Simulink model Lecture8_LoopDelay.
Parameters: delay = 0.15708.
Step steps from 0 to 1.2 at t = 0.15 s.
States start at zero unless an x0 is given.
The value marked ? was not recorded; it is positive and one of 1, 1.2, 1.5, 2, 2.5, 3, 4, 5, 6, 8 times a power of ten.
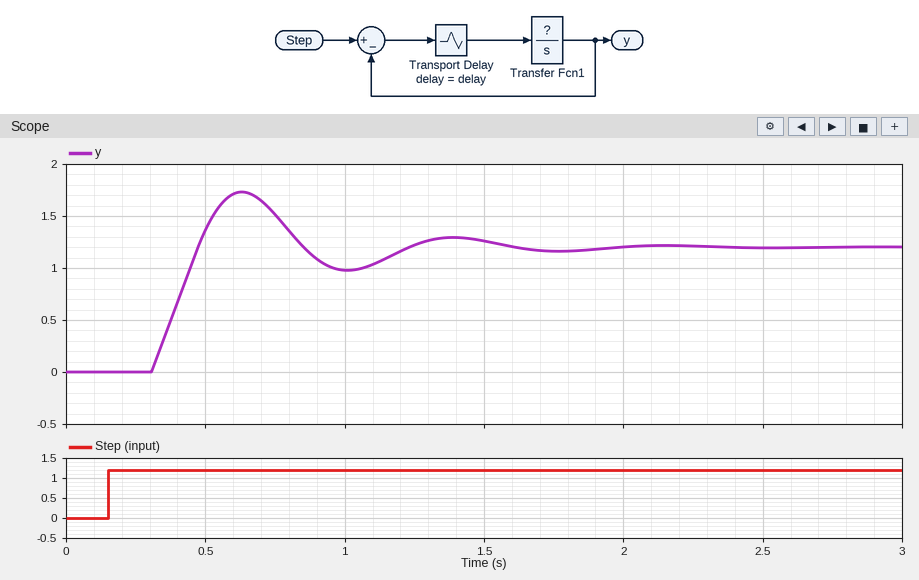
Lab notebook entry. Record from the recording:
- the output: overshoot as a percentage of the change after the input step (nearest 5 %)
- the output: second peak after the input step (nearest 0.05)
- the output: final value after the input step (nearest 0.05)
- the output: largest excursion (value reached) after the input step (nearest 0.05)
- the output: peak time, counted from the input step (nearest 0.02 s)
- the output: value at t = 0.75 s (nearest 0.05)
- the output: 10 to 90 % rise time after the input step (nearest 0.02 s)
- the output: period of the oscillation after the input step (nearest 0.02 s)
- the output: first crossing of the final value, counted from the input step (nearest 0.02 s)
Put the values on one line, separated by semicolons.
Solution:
45 %; 1.30; 1.20; 1.75; 0.48 s; 1.50; 0.14 s; 0.76 s; 0.32 s
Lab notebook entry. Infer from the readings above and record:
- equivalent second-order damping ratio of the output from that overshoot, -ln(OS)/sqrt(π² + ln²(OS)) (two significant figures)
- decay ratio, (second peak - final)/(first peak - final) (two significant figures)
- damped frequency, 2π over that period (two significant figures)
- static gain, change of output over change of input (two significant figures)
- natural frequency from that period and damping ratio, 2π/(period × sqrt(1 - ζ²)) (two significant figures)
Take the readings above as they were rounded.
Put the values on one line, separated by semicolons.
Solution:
0.25; 0.18; 8.3 rad/s; 1.0; 8.5 rad/s
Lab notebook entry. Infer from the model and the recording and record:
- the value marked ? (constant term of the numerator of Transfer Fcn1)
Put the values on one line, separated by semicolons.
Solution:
6
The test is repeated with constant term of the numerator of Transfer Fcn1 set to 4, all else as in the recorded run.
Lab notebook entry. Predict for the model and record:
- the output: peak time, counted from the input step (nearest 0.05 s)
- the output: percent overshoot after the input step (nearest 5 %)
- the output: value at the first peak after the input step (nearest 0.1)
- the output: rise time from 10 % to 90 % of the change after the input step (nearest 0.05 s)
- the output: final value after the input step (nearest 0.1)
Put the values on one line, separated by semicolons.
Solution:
0.60 s; 15 %; 1.4; 0.20 s; 1.2
